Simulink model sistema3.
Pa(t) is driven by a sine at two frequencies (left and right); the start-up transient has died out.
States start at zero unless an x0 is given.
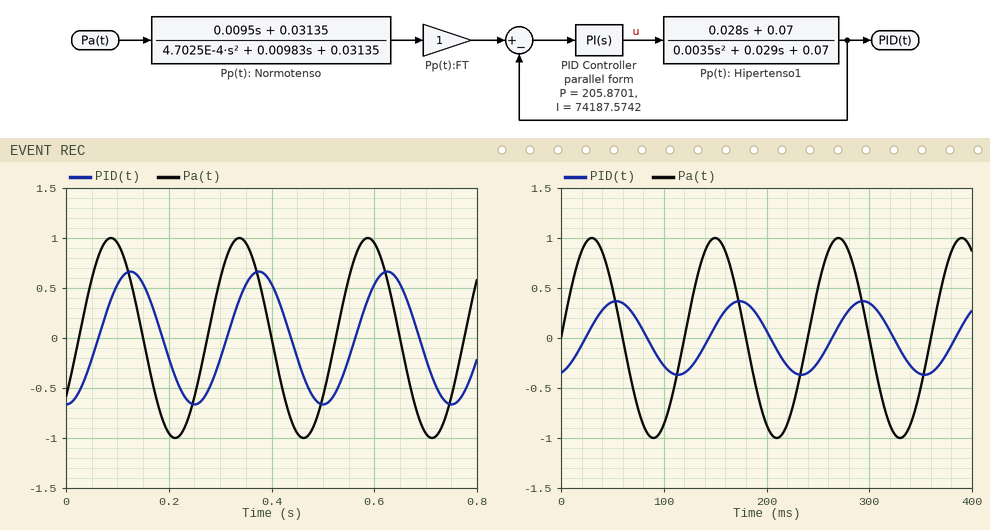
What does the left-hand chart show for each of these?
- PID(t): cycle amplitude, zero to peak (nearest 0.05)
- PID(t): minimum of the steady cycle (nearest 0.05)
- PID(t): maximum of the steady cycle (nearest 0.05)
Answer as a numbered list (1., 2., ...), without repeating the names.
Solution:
1. 0.65
2. -0.65
3. 0.65
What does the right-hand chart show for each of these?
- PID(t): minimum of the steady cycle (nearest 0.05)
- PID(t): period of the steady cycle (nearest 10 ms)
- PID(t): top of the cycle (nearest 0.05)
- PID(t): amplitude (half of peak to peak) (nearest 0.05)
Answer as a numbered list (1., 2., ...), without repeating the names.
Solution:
1. -0.35
2. 120 ms
3. 0.35
4. 0.35
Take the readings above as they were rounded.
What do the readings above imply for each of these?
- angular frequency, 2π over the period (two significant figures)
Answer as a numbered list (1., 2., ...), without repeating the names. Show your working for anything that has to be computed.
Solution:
1. 2π / 120 = 0.052 rad/ms
